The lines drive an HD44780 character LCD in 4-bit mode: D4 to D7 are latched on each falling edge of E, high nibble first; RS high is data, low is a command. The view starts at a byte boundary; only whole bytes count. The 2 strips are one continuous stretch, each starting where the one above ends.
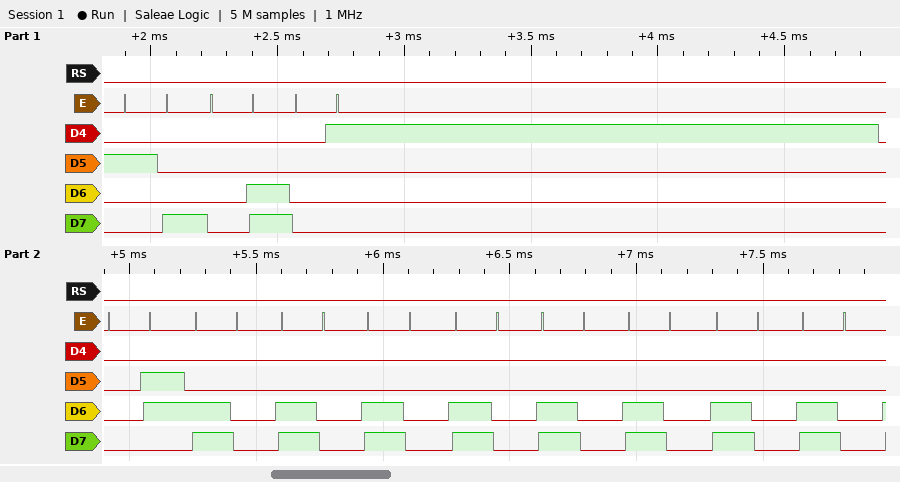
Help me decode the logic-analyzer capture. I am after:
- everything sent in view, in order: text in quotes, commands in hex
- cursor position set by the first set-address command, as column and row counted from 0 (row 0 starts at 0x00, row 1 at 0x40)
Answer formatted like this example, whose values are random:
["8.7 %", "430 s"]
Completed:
["0x28 0x0C 0x01 0x06 0xC0 0xC0 0xC0 0xC0 0xC0 0xC0 0xC0 0xC0", "column 0, row 1"]
